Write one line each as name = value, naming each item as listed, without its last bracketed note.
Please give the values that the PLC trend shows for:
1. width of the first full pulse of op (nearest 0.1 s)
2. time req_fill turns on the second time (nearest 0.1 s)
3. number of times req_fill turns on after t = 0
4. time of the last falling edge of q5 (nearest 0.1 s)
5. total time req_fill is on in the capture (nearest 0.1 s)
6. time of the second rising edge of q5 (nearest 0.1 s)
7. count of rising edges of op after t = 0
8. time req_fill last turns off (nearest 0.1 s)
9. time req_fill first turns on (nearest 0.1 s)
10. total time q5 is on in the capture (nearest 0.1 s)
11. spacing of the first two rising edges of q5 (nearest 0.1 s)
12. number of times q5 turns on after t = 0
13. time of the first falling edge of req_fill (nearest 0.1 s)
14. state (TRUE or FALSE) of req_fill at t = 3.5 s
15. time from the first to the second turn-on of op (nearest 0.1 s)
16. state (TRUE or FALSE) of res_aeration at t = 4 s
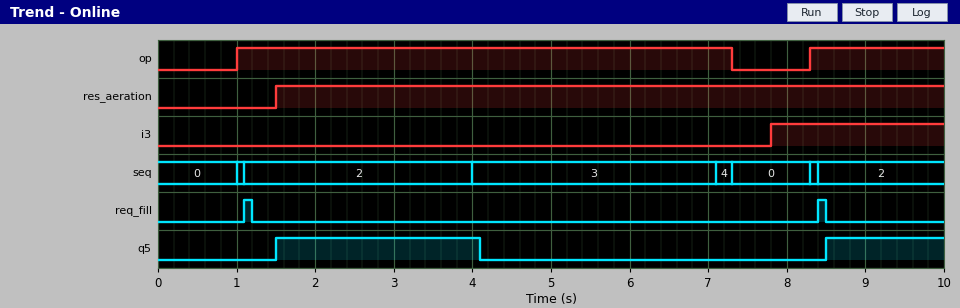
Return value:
width of the first full pulse of op = 6.3 s
time req_fill turns on the second time = 8.4 s
number of times req_fill turns on after t = 0 = 2
time of the last falling edge of q5 = 4.1 s
total time req_fill is on in the capture = 0.2 s
time of the second rising edge of q5 = 8.5 s
count of rising edges of op after t = 0 = 2
time req_fill last turns off = 8.5 s
time req_fill first turns on = 1.1 s
total time q5 is on in the capture = 4.1 s
spacing of the first two rising edges of q5 = 7.0 s
number of times q5 turns on after t = 0 = 2
time of the first falling edge of req_fill = 1.2 s
state (TRUE or FALSE) of req_fill at t = 3.5 s = FALSE
time from the first to the second turn-on of op = 7.3 s
state (TRUE or FALSE) of res_aeration at t = 4 s = TRUE
